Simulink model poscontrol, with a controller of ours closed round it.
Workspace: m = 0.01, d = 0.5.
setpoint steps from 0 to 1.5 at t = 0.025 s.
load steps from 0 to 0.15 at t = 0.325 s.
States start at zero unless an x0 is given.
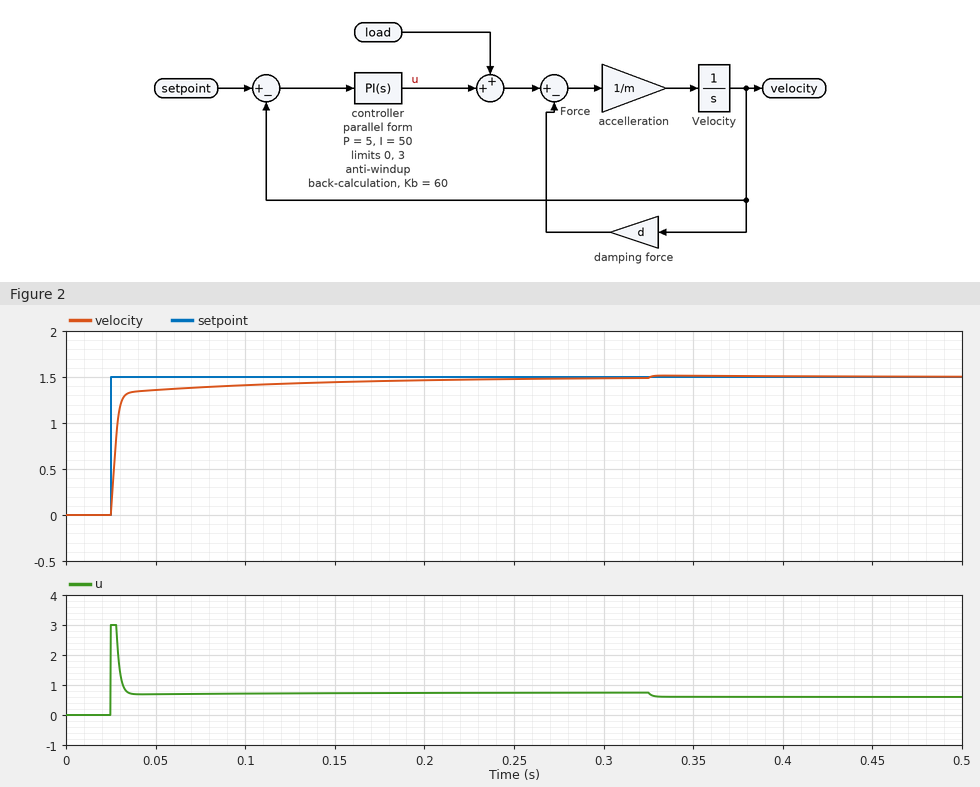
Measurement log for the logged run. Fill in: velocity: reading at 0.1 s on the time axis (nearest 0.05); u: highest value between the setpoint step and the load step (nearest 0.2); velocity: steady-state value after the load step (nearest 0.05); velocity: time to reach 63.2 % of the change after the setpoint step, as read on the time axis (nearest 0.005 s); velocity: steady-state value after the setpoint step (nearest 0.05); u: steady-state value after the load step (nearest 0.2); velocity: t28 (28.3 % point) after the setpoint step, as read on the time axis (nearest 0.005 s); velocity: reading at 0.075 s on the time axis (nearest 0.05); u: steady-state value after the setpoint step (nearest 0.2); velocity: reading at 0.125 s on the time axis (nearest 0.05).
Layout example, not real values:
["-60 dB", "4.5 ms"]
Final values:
["1.40", "3.0", "1.50", "0.030 s", "1.50", "0.6", "0.025 s", "1.40", "0.8", "1.45"]
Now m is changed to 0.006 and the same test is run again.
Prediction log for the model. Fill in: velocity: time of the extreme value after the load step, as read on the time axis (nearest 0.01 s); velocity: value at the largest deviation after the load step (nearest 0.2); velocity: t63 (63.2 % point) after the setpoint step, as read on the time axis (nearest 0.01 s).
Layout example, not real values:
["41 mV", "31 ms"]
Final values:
["0.33 s", "1.6", "0.03 s"]
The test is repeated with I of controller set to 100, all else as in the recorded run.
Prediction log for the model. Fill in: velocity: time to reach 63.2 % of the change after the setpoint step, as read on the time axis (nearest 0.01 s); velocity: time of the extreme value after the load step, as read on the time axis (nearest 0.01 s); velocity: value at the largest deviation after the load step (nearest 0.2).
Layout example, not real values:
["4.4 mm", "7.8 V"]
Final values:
["0.03 s", "0.33 s", "1.6"]
